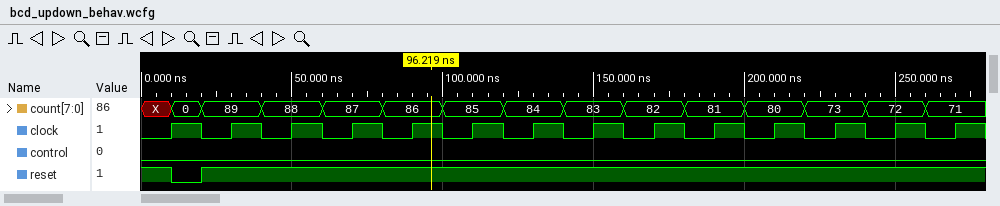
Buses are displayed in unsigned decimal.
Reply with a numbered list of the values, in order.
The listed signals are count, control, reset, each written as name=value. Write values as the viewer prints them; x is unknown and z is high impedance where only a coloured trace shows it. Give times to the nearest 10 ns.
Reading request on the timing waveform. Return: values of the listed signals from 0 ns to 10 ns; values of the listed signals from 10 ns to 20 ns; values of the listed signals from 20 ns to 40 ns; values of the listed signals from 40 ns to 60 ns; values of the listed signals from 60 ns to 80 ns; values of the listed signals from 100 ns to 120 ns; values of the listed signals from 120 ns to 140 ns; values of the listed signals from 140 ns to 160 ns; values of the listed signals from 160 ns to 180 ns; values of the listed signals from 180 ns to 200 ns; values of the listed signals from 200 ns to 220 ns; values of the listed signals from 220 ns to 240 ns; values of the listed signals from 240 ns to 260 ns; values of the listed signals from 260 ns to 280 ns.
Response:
1. count=X, control=0, reset=1
2. count=0, control=0, reset=0
3. count=89, control=0, reset=1
4. count=88, control=0, reset=1
5. count=87, control=0, reset=1
6. count=85, control=0, reset=1
7. count=84, control=0, reset=1
8. count=83, control=0, reset=1
9. count=82, control=0, reset=1
10. count=81, control=0, reset=1
11. count=80, control=0, reset=1
12. count=73, control=0, reset=1
13. count=72, control=0, reset=1
14. count=71, control=0, reset=1
